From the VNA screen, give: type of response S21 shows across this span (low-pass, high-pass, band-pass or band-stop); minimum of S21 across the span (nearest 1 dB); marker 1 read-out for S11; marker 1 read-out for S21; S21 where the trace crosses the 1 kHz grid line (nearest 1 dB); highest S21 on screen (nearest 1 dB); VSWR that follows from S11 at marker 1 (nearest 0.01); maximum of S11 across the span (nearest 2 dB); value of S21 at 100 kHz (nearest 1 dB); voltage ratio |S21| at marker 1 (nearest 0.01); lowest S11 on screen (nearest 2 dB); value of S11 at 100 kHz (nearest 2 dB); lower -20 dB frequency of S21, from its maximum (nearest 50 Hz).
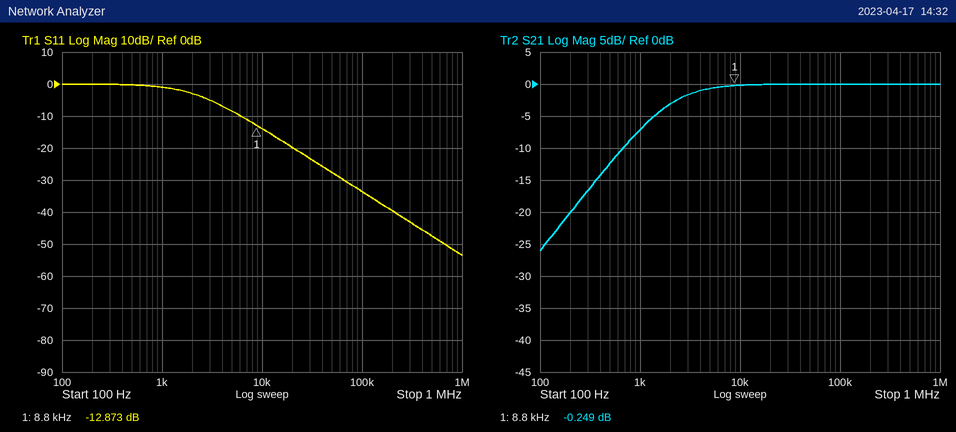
high-pass
-26 dB
-12.873 dB
-0.249 dB
-7 dB
0 dB
1.59
0 dB
0 dB
0.97
-54 dB
-34 dB
200 Hz
